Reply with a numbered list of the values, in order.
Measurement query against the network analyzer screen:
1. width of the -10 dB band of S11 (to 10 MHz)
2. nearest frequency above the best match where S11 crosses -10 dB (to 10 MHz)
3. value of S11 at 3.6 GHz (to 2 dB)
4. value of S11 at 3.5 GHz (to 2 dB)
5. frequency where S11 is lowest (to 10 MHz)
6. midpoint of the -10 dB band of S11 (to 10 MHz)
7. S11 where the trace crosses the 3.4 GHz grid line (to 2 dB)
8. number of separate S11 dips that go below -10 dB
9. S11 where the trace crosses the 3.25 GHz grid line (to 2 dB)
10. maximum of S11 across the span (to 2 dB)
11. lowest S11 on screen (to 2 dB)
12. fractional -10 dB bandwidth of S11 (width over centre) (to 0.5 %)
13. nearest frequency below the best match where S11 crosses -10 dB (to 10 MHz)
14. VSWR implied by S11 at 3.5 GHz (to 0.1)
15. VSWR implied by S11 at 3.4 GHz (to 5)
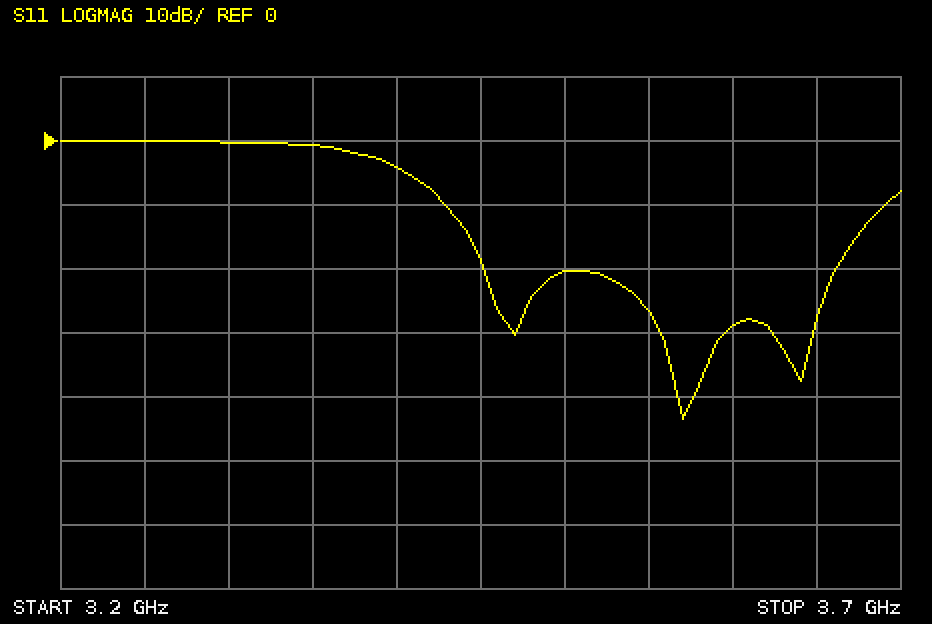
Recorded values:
1. 260 MHz
2. 3.69 GHz
3. -28 dB
4. -20 dB
5. 3.57 GHz
6. 3.56 GHz
7. -4 dB
8. 3
9. 0 dB
10. 0 dB
11. -44 dB
12. 7.5 %
13. 3.43 GHz
14. 1.2
15. 5
